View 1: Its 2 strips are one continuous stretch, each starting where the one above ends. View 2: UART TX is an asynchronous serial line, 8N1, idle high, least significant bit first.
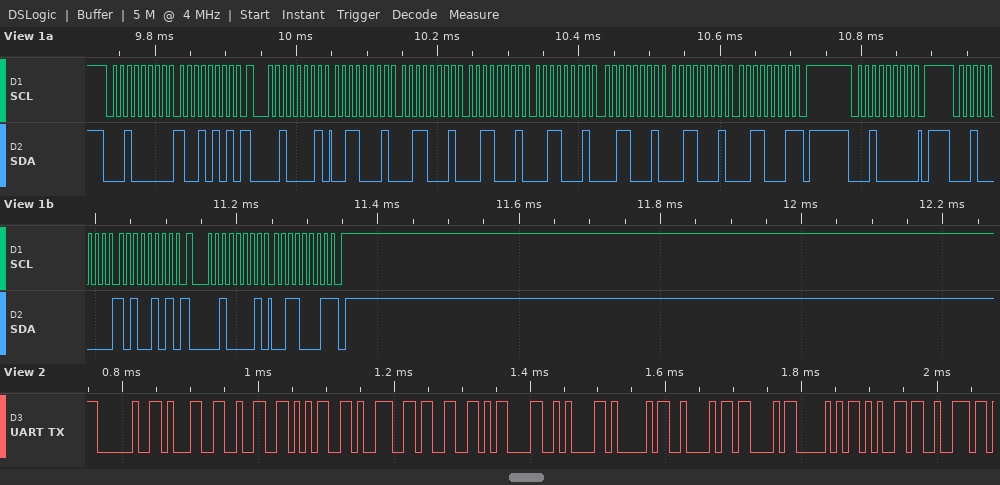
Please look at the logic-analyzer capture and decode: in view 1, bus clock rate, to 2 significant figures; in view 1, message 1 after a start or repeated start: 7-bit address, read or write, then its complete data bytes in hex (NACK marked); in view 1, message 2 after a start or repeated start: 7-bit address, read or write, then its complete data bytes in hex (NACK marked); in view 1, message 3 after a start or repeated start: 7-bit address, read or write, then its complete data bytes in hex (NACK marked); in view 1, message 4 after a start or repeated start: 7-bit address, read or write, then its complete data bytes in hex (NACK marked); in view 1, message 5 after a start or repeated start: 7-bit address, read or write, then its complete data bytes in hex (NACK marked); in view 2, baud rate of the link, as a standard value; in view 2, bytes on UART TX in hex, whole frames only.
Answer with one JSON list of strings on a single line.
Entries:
["100 kHz", "0x10 write: 95", "0x10 read: 31 31 31 31 31 31 31 NACK", "0x10 write", "0x10 write: A5", "0x10 read: 31 NACK", "115200 baud", "0x20 0x31 0x32 0x35 0x39 0x33 0x0D 0x0A 0x41 0x42 0x43 0x50 0x65 0x72"]
